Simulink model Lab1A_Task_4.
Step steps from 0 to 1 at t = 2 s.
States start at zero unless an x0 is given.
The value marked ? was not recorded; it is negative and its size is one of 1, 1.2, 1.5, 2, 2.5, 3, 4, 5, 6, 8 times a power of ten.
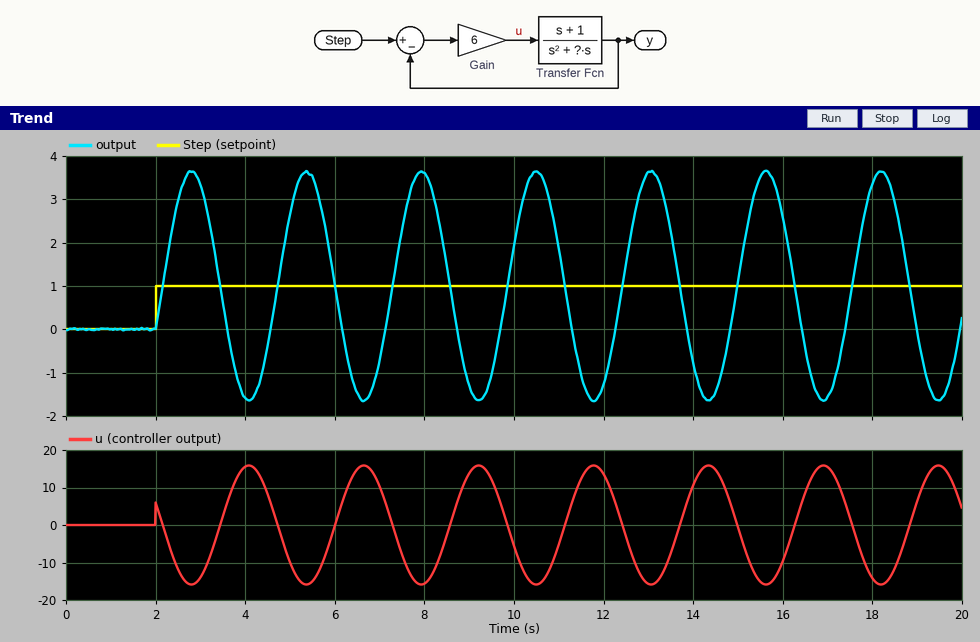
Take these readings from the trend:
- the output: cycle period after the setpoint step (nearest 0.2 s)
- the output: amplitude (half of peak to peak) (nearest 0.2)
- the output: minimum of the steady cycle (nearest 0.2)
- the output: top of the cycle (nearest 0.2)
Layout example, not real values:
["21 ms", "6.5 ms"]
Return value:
["2.6 s", "2.6", "-1.6", "3.6"]
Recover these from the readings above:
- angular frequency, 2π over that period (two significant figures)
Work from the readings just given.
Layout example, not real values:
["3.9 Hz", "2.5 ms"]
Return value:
["2.4 rad/s"]
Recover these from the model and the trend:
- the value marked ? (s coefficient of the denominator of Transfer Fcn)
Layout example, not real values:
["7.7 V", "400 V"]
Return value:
["-6"]
